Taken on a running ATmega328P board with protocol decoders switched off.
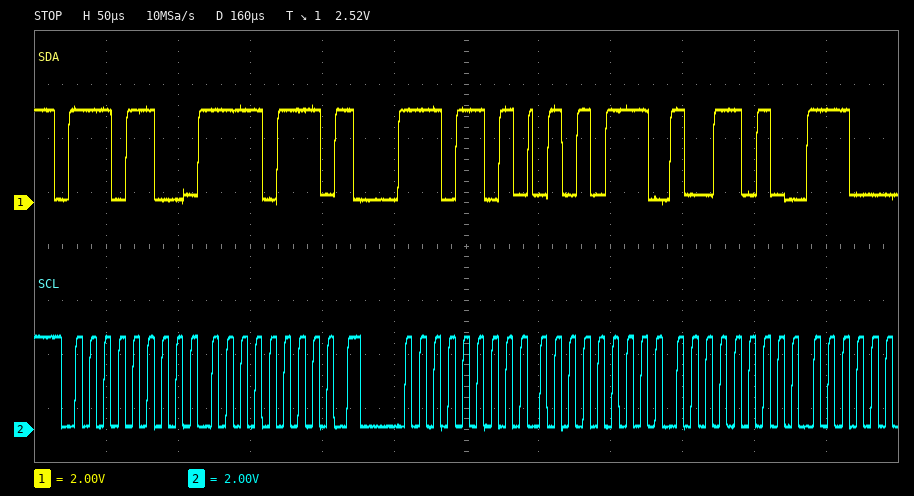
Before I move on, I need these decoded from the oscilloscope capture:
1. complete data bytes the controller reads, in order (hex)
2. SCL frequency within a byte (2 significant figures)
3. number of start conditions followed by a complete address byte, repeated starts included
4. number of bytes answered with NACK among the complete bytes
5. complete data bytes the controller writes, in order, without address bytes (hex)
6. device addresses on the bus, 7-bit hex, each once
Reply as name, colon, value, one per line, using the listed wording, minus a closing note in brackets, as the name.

complete data bytes the controller reads, in order: 57 9A
SCL frequency within a byte: 100 kHz
number of start conditions followed by a complete address byte, repeated starts included: 2
number of bytes answered with NACK among the complete bytes: 0
complete data bytes the controller writes, in order, without address bytes: F7
device addresses on the bus, 7-bit hex, each once: 0x76
